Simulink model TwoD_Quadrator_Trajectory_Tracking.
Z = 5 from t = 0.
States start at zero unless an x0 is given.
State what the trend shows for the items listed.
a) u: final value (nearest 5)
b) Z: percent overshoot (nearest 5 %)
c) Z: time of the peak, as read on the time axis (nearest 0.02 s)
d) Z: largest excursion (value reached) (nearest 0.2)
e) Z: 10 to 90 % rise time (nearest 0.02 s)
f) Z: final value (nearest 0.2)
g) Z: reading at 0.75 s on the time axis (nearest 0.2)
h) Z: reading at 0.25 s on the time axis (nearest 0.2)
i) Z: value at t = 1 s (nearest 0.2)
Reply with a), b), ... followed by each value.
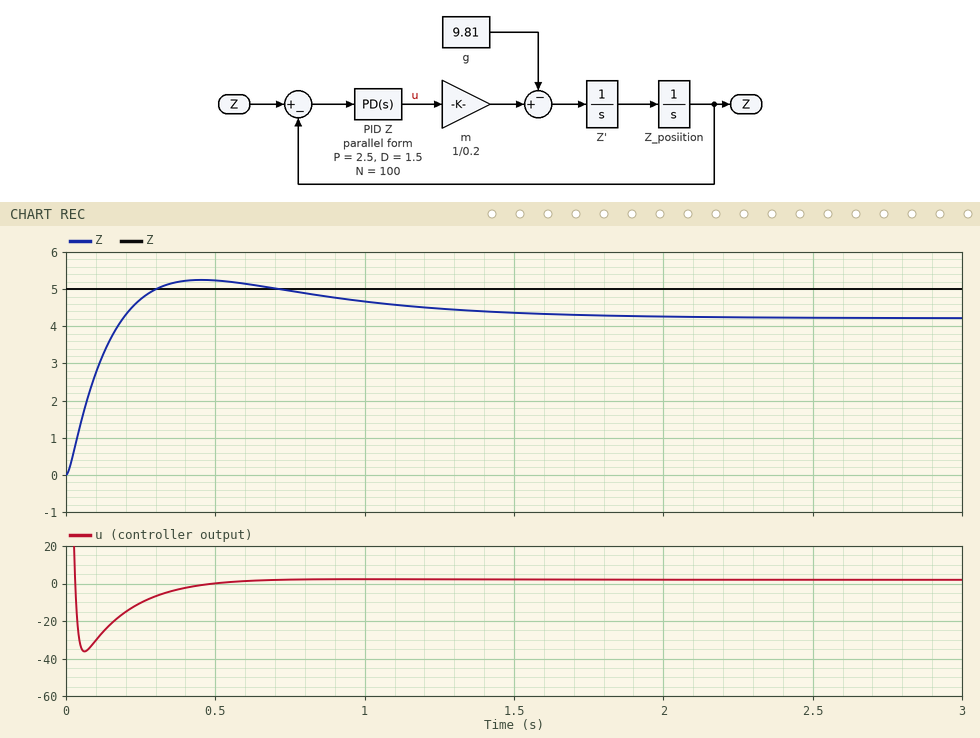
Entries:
a) 0
b) 25 %
c) 0.46 s
d) 5.2
e) 0.14 s
f) 4.2
g) 5.0
h) 4.8
i) 4.6
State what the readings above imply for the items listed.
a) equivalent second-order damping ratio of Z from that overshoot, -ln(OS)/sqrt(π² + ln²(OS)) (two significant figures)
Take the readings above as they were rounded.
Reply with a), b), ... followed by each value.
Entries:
a) 0.40
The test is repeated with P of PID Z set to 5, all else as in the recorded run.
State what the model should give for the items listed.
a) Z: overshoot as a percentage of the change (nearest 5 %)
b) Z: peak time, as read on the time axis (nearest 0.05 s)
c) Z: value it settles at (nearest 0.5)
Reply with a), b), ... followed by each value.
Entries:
a) 25 %
b) 0.40 s
c) 4.5
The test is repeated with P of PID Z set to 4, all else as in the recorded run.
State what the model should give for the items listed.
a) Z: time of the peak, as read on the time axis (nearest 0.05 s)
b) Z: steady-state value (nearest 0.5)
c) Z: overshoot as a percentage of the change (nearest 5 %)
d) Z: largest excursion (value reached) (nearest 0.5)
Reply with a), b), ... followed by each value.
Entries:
a) 0.40 s
b) 4.5
c) 25 %
d) 5.5
